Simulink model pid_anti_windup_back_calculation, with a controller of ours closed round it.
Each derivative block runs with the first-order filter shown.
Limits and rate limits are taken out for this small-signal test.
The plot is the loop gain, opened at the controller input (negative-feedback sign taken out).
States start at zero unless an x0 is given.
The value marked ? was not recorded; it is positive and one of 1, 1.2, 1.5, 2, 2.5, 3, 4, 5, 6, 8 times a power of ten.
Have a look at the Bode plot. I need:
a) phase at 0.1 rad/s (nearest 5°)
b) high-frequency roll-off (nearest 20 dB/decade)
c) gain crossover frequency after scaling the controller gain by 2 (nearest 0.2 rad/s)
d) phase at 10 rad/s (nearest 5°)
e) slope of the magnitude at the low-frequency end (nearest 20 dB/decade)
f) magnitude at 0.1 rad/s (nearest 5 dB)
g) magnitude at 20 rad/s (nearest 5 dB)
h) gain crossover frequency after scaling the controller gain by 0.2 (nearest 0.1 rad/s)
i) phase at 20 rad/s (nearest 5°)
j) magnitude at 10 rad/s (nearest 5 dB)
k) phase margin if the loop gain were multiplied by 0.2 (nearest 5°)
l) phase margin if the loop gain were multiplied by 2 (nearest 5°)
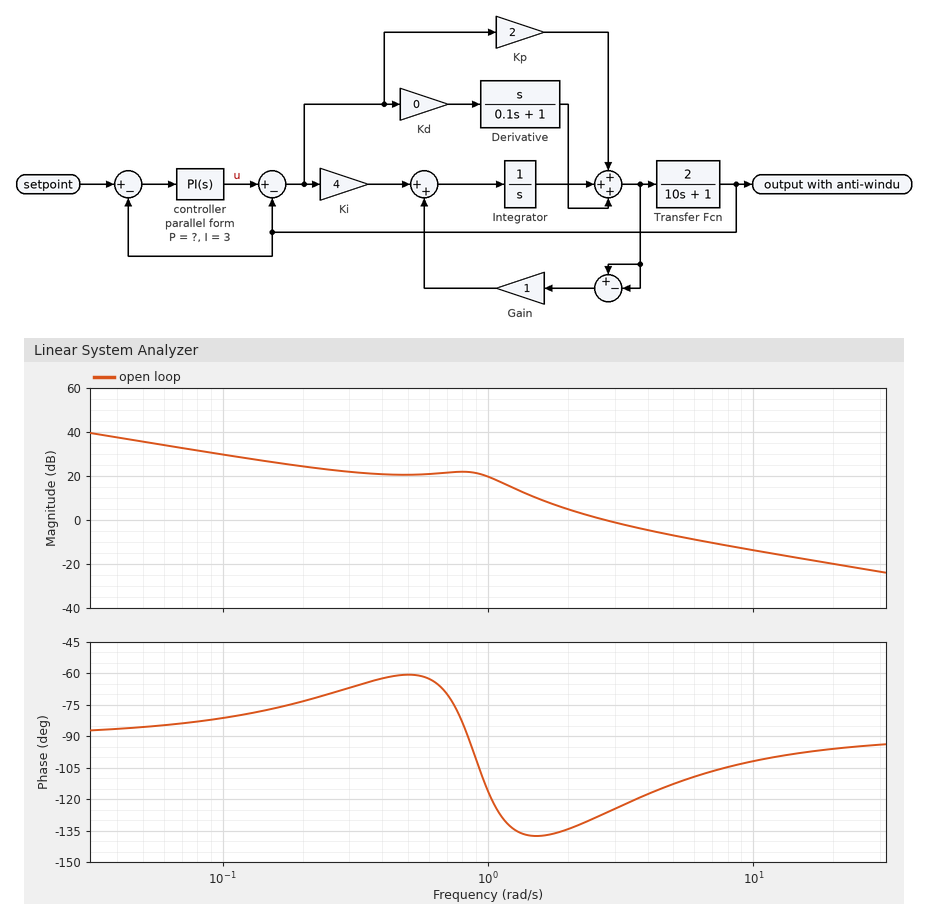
-80°
-20 dB/decade
4.6 rad/s
-100°
-20 dB/decade
30 dB
-20 dB
1.3 rad/s
-95°
-15 dB
45°
65°
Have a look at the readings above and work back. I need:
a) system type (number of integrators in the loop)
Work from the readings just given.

1
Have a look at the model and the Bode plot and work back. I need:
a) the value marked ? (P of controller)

5
